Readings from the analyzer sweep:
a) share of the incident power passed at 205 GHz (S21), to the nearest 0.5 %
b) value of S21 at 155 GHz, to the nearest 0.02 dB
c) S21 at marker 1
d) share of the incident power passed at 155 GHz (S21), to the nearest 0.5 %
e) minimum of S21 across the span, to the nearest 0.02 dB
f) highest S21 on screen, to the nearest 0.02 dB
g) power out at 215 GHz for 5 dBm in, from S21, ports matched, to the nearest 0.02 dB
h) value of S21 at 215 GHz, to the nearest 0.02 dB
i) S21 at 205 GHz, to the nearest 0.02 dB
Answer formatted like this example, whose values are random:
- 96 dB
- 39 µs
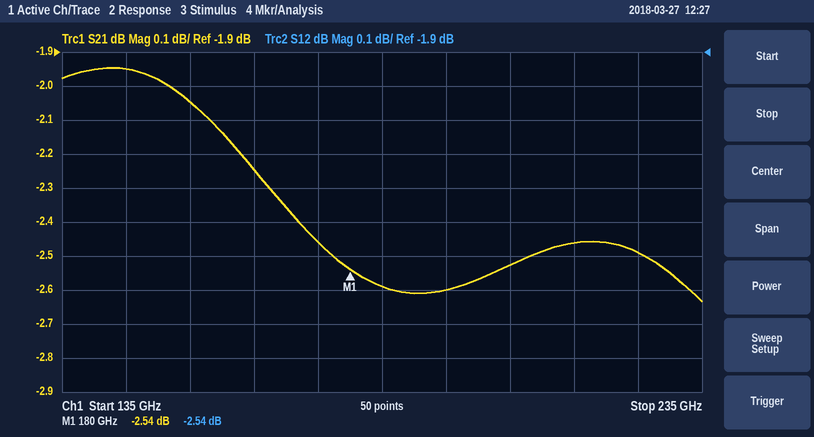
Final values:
- 56.0 %
- -2.04 dB
- -2.54 dB
- 62.5 %
- -2.64 dB
- -1.94 dB
- 2.54 dBm
- -2.46 dB
- -2.52 dB
